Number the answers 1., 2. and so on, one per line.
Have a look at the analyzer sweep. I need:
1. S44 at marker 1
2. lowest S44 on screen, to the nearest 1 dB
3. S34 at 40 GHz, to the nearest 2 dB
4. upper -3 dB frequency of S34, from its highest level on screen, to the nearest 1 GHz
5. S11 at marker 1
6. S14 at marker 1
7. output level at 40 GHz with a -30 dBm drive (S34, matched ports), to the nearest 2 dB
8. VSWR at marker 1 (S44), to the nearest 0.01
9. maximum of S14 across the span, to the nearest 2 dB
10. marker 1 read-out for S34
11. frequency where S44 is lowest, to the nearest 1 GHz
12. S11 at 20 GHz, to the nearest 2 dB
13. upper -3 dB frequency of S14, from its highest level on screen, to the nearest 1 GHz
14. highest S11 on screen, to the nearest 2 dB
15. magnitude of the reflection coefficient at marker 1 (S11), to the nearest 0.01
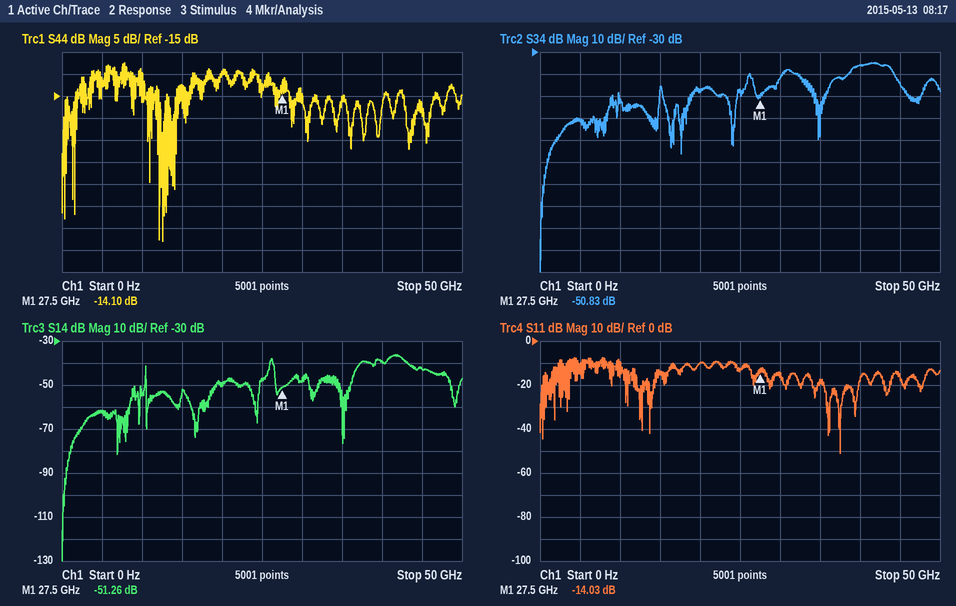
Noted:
1. -14.10 dB
2. -48 dB
3. -36 dB
4. 44 GHz
5. -14.03 dB
6. -51.26 dB
7. -66 dBm
8. 1.49
9. -36 dB
10. -50.83 dB
11. 13 GHz
12. -10 dB
13. 43 GHz
14. -8 dB
15. 0.20
